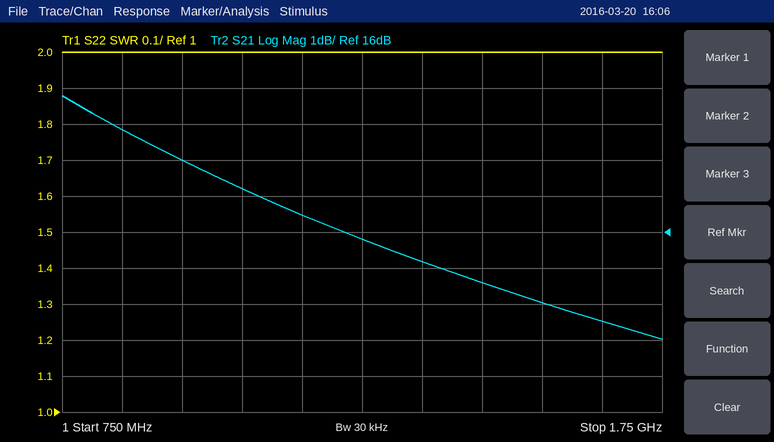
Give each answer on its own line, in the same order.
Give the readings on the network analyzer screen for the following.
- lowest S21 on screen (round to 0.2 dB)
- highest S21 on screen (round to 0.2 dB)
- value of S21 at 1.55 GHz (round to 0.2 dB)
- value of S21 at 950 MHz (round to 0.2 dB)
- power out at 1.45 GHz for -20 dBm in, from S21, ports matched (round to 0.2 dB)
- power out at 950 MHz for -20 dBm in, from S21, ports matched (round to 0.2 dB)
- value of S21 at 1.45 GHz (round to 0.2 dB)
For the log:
13.0 dB
19.8 dB
14.0 dB
18.0 dB
-5.4 dBm
-2.0 dBm
14.6 dB
